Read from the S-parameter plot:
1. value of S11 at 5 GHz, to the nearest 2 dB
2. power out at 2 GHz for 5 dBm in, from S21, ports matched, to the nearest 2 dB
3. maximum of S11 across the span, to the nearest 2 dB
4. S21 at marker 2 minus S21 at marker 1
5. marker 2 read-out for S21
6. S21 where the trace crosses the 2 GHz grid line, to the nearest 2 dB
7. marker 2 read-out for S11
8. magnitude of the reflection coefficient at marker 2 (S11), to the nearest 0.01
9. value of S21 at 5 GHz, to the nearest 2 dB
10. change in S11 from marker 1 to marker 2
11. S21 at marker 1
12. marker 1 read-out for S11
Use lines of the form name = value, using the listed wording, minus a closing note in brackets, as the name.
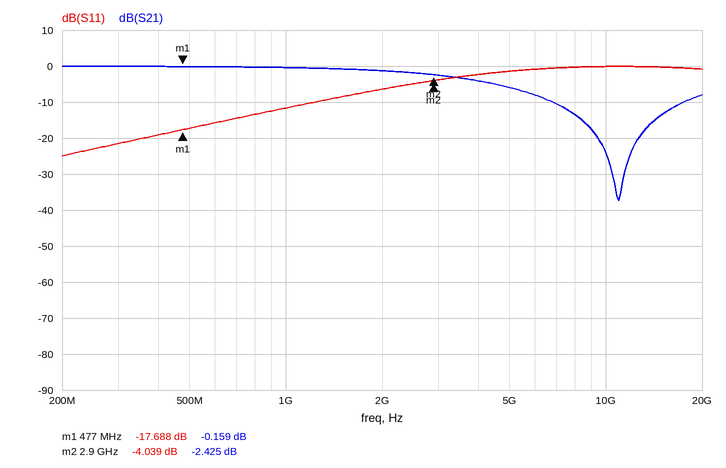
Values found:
value of S11 at 5 GHz, to the nearest 2 dB = -2 dB
power out at 2 GHz for 5 dBm in, from S21, ports matched, to the nearest 2 dB = 4 dBm
maximum of S11 across the span, to the nearest 2 dB = 0 dB
S21 at marker 2 minus S21 at marker 1 = -2.266 dB
marker 2 read-out for S21 = -2.425 dB
S21 where the trace crosses the 2 GHz grid line, to the nearest 2 dB = -2 dB
marker 2 read-out for S11 = -4.039 dB
magnitude of the reflection coefficient at marker 2 (S11), to the nearest 0.01 = 0.63
value of S21 at 5 GHz, to the nearest 2 dB = -6 dB
change in S11 from marker 1 to marker 2 = 13.649 dB
S21 at marker 1 = -0.159 dB
marker 1 read-out for S11 = -17.688 dB
